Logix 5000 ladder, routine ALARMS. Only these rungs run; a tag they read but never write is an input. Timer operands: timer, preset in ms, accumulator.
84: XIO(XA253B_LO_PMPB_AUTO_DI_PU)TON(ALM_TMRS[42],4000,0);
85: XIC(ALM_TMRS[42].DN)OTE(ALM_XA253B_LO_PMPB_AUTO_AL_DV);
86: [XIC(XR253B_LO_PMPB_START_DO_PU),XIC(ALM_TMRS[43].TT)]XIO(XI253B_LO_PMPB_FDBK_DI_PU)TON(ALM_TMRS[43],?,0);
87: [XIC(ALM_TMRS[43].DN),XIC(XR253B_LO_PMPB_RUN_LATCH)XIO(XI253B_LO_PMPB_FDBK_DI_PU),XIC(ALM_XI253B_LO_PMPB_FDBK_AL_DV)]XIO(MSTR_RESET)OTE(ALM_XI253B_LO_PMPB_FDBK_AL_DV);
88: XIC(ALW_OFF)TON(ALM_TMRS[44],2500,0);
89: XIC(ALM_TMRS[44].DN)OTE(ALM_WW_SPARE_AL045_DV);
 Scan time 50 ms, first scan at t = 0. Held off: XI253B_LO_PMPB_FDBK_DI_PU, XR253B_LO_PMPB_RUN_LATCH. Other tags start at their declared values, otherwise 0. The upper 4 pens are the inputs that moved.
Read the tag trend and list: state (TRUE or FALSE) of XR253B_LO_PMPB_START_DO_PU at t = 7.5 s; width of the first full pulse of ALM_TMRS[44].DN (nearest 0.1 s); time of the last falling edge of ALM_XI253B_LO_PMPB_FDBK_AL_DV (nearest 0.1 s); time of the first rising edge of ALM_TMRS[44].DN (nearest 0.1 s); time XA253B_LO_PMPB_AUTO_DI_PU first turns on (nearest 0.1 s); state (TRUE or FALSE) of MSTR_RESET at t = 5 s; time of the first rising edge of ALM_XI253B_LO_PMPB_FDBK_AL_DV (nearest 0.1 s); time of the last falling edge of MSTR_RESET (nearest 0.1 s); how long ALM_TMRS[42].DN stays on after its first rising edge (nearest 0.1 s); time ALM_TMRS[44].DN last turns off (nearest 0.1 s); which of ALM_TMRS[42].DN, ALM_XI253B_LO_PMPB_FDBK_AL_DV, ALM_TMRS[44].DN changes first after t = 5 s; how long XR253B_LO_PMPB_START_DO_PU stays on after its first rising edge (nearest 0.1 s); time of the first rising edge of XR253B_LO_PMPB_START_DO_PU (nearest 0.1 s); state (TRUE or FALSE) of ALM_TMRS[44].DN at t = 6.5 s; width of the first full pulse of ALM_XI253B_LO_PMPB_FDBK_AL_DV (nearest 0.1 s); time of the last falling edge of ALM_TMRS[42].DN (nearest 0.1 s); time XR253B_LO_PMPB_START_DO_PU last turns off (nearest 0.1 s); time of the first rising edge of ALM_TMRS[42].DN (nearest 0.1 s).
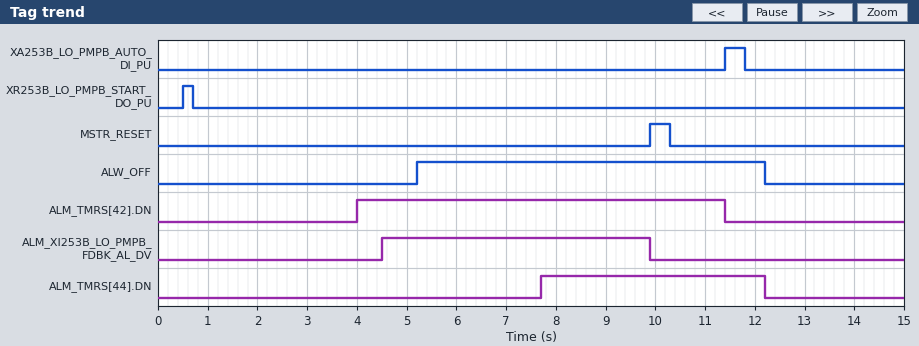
FALSE
4.5 s
9.9 s
7.7 s
11.4 s
FALSE
4.5 s
10.3 s
7.4 s
12.2 s
ALM_TMRS[44].DN
0.2 s
0.5 s
FALSE
5.4 s
11.4 s
0.7 s
4.0 s
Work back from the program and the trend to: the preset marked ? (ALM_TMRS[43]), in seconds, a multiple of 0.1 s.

4.0 s
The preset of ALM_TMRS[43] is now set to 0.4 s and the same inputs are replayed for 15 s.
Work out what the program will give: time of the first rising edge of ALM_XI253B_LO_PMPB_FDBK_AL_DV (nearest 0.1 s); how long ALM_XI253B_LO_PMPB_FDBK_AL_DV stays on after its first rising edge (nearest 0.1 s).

0.9 s
9.0 s
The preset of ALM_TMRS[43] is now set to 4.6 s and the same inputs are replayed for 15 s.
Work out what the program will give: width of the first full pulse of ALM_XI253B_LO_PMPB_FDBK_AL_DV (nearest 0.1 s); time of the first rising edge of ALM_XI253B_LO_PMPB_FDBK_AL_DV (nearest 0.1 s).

4.8 s
5.1 s
